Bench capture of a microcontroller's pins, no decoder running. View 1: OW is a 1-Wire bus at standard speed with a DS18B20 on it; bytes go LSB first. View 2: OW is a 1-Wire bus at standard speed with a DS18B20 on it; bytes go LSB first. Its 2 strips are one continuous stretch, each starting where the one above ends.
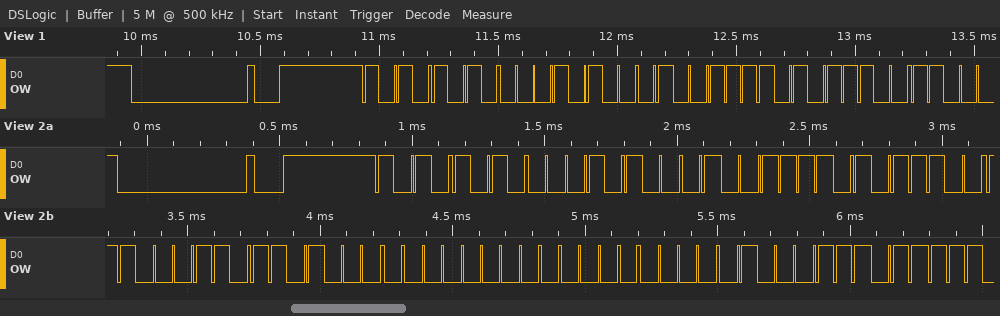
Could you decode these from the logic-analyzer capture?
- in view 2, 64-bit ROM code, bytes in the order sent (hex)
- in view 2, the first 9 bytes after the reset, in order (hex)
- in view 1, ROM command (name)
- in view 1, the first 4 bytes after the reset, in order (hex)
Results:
28 F2 3A 63 0B 00 00 E2
55 28 F2 3A 63 0B 00 00 E2
Match ROM
55 28 F2 3A
